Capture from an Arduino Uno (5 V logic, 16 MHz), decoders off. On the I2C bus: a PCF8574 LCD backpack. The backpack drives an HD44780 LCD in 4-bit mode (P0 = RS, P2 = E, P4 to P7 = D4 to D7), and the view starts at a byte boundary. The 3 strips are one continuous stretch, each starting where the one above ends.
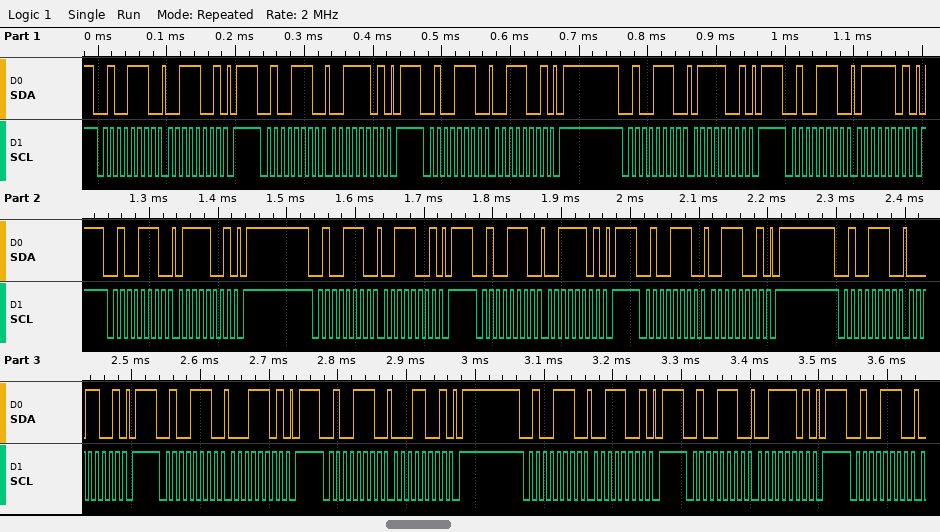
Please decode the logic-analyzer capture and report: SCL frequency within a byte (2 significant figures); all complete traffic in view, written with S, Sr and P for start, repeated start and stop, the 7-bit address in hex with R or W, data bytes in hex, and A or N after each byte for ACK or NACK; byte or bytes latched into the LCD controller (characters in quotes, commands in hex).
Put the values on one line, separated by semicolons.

100 kHz; S 27W A 39 A P S 27W A 3D A P S 27W A 39 A P S 27W A 79 A P S 27W A 7D A P S 27W A 79 A P S 27W A 39 A P S 27W A 3D A P S 27W A 39 A P S 27W A 19 A P S 27W A 1D A P S 27W A 19 A P S 27W A 39 A P S 27W A 3D A P S 27W A; '7' '1'
